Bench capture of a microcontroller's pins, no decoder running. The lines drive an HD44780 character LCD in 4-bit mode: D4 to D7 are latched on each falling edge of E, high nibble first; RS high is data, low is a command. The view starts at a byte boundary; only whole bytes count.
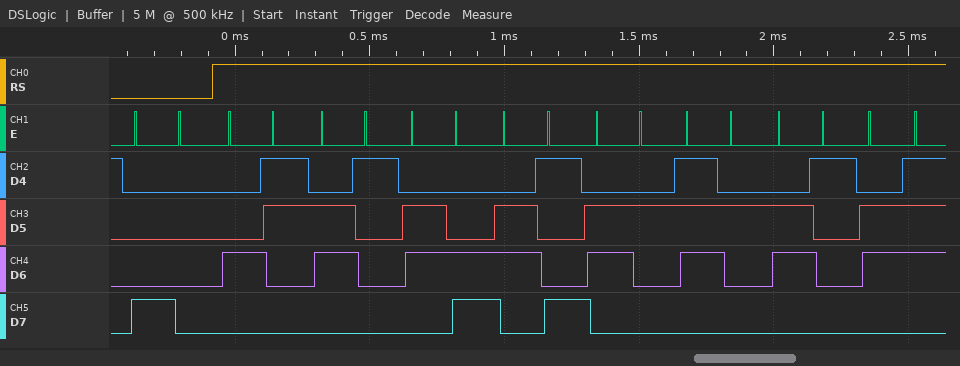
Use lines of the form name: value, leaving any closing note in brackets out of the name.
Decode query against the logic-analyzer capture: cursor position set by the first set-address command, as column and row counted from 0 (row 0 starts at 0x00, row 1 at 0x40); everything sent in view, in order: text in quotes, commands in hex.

cursor position set by the first set-address command, as column and row counted from 0: column 0, row 0
everything sent in view, in order: text in quotes, commands in hex: 0x80 "Calibrag"
